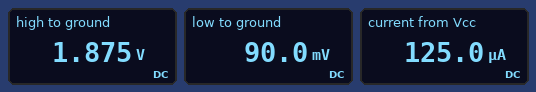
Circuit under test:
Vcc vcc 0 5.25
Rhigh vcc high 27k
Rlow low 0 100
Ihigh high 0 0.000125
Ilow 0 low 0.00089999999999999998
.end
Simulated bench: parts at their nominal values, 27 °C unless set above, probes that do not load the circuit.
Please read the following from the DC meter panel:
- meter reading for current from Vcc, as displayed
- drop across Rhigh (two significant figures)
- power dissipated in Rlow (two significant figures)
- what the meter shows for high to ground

125.0 µA
3.4 V
81 µW
1.875 V
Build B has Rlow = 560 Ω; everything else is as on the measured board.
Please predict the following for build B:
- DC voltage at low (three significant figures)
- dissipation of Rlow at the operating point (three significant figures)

504 mV
454 µW
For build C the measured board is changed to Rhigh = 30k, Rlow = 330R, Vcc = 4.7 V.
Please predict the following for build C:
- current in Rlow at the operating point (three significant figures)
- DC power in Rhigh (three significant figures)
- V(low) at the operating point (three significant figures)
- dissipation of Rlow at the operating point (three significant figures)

900 µA
469 µW
297 mV
267 µW
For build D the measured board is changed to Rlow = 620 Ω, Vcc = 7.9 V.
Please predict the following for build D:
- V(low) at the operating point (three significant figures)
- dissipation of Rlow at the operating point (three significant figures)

558 mV
502 µW
